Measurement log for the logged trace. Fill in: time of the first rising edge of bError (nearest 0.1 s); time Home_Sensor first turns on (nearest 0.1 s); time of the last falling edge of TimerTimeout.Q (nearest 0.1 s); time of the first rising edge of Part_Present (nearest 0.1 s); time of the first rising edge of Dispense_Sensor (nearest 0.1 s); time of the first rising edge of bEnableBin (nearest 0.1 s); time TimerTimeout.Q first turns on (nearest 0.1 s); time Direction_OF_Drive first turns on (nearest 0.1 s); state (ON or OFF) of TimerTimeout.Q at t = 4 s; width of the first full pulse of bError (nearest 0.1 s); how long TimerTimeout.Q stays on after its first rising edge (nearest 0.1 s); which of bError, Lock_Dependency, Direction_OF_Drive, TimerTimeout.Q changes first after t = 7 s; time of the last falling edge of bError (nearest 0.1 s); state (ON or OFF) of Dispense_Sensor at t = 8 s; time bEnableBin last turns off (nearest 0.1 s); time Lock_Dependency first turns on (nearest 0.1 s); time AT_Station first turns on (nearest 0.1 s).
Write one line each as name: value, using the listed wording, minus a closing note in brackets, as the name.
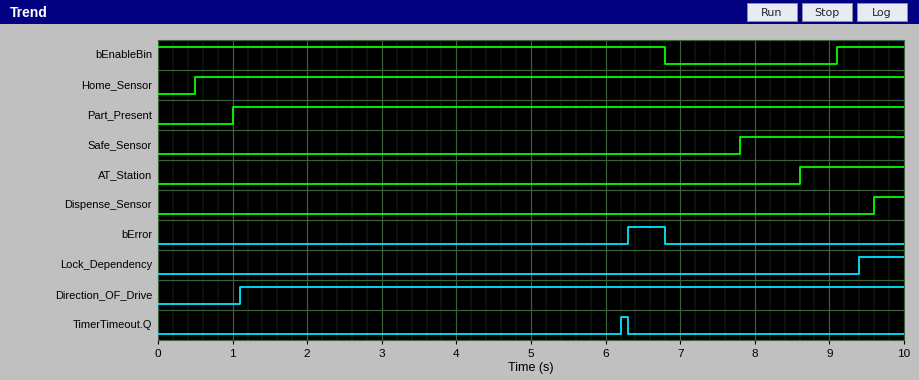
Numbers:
time of the first rising edge of bError: 6.3 s
time Home_Sensor first turns on: 0.5 s
time of the last falling edge of TimerTimeout.Q: 6.3 s
time of the first rising edge of Part_Present: 1.0 s
time of the first rising edge of Dispense_Sensor: 9.6 s
time of the first rising edge of bEnableBin: 9.1 s
time TimerTimeout.Q first turns on: 6.2 s
time Direction_OF_Drive first turns on: 1.1 s
state (ON or OFF) of TimerTimeout.Q at t = 4 s: OFF
width of the first full pulse of bError: 0.5 s
how long TimerTimeout.Q stays on after its first rising edge: 0.1 s
which of bError, Lock_Dependency, Direction_OF_Drive, TimerTimeout.Q changes first after t = 7 s: Lock_Dependency
time of the last falling edge of bError: 6.8 s
state (ON or OFF) of Dispense_Sensor at t = 8 s: OFF
time bEnableBin last turns off: 6.8 s
time Lock_Dependency first turns on: 9.4 s
time AT_Station first turns on: 8.6 s
